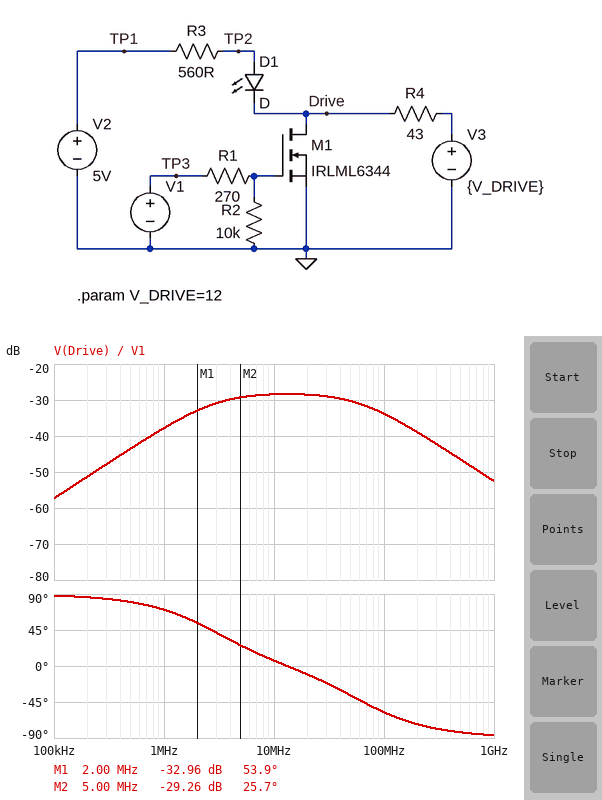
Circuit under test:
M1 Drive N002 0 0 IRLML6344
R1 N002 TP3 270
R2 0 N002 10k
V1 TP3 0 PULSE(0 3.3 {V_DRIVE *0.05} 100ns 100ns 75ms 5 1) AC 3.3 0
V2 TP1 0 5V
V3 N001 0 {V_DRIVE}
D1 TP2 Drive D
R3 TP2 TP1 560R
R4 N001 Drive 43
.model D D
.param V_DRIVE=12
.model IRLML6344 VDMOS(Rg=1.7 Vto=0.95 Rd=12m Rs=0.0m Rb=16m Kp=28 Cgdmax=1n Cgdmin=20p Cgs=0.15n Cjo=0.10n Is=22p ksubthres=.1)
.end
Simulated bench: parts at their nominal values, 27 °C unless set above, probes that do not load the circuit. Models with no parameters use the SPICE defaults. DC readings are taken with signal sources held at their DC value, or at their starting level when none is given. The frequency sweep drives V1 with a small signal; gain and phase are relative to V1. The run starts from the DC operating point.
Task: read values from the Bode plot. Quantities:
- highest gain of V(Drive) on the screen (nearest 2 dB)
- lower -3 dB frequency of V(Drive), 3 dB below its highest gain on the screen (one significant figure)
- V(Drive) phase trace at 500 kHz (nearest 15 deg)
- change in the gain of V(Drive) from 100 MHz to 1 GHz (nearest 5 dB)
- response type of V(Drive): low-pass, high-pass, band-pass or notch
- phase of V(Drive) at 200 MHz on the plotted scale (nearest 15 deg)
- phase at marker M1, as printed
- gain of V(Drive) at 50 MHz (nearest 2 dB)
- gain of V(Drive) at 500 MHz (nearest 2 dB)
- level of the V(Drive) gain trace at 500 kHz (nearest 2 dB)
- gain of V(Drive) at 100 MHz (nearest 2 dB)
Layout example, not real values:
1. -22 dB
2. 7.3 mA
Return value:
1. -28 dB
2. 3 MHz
3. 75 deg
4. -20 dB
5. band-pass
6. -75 deg
7. 53.9 deg
8. -30 dB
9. -46 dB
10. -44 dB
11. -34 dB
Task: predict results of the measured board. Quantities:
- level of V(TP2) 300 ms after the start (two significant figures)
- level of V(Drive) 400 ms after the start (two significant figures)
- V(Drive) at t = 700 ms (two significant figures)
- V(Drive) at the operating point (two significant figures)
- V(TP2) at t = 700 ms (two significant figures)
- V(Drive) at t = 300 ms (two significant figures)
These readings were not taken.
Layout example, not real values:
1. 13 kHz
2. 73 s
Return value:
1. 5.0 V
2. 12 V
3. 12 V
4. 12 V
5. 5.0 V
6. 12 V
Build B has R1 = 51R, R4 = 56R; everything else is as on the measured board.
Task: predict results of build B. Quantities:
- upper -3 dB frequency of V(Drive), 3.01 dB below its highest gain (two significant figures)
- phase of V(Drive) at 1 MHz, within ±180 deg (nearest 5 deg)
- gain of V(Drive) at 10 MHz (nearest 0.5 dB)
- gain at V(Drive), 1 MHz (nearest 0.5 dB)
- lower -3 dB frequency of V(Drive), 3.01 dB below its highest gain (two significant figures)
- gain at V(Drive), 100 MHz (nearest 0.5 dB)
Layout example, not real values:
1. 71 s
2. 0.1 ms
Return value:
1. 72 MHz
2. 85 deg
3. -17.0 dB
4. -35.0 dB
5. 9.3 MHz
6. -19.5 dB
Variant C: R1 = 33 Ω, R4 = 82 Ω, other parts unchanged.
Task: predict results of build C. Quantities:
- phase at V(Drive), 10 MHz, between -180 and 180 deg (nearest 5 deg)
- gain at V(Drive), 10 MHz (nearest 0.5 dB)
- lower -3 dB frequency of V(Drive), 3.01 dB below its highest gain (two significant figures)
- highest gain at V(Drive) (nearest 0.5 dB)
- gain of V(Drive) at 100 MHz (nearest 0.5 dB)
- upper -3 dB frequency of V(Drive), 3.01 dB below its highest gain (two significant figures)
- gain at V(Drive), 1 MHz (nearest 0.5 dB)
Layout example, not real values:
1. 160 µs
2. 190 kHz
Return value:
1. 45 deg
2. -13.0 dB
3. 10 MHz
4. -10.0 dB
5. -15.5 dB
6. 68 MHz
7. -31.5 dB
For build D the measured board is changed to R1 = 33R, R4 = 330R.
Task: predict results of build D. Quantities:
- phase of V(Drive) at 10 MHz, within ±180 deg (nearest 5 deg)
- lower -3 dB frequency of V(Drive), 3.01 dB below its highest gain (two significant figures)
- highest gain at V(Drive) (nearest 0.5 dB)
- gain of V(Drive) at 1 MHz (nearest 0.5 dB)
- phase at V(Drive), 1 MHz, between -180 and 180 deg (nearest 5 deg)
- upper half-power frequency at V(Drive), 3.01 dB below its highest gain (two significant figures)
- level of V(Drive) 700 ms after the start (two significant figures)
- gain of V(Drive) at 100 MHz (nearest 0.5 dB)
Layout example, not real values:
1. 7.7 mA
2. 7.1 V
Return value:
1. 10 deg
2. 4.4 MHz
3. -5.5 dB
4. -19.5 dB
5. 80 deg
6. 40 MHz
7. 12 V
8. -15.0 dB
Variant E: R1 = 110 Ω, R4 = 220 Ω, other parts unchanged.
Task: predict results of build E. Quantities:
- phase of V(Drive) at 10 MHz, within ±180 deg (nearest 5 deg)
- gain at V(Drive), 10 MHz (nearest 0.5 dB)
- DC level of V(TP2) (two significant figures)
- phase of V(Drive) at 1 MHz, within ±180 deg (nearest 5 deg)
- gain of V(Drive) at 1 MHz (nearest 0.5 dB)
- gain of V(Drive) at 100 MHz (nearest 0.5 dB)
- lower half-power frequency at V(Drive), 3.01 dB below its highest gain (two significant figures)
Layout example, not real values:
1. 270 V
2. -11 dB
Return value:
1. -5 deg
2. -11.0 dB
3. 5.0 V
4. 75 deg
5. -23.0 dB
6. -25.0 dB
7. 3.5 MHz
